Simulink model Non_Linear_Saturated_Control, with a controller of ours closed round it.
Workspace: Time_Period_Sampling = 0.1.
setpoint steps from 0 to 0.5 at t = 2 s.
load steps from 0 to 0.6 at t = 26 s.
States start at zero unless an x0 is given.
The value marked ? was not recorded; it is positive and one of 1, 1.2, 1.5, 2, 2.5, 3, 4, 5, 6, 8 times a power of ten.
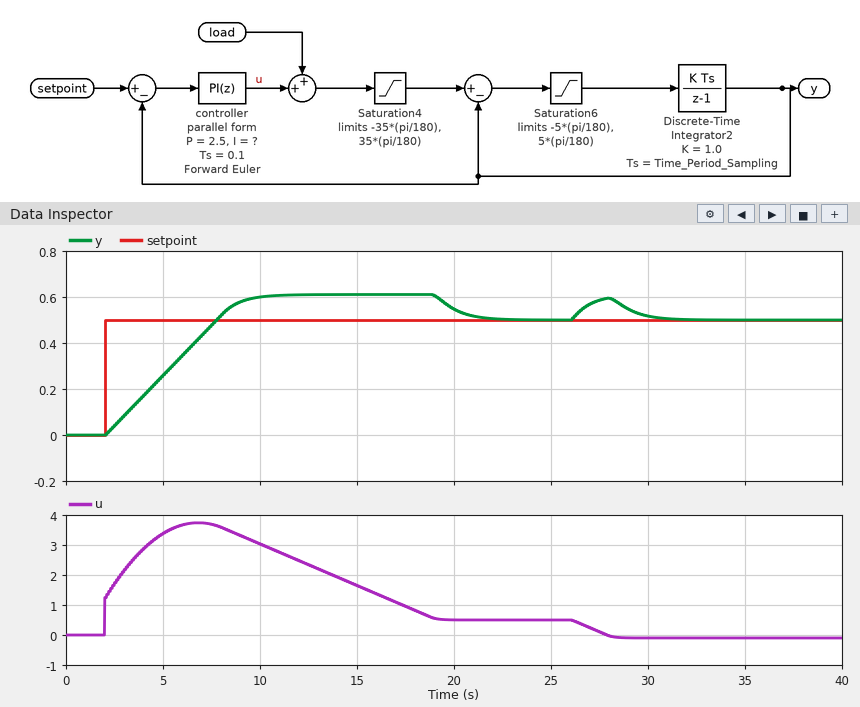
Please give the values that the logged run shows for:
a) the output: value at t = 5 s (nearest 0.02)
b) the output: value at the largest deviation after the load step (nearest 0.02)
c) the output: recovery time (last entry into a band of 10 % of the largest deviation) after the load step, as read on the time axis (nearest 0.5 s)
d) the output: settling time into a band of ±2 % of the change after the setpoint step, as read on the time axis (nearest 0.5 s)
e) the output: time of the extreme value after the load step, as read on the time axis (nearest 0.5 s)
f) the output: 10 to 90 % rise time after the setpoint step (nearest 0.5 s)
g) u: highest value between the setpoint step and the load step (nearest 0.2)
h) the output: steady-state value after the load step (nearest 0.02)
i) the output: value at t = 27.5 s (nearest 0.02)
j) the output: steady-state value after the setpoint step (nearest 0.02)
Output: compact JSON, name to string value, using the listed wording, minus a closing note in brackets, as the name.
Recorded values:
{"the output: value at t = 5 s": "0.26", "the output: value at the largest deviation after the load step": "0.60", "the output: recovery time (last entry into a band of 10 % of the largest deviation) after the load step, as read on the time axis": "30.5 s", "the output: settling time into a band of ±2 % of the change after the setpoint step, as read on the time axis": "21.5 s", "the output: time of the extreme value after the load step, as read on the time axis": "28.0 s", "the output: 10 to 90 % rise time after the setpoint step": "4.5 s", "u: highest value between the setpoint step and the load step": "3.8", "the output: steady-state value after the load step": "0.50", "the output: value at t = 27.5 s": "0.58", "the output: steady-state value after the setpoint step": "0.50"}
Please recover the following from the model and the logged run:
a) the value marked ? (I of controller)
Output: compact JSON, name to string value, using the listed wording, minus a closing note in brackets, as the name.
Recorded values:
{"the value marked ?": "2.5"}
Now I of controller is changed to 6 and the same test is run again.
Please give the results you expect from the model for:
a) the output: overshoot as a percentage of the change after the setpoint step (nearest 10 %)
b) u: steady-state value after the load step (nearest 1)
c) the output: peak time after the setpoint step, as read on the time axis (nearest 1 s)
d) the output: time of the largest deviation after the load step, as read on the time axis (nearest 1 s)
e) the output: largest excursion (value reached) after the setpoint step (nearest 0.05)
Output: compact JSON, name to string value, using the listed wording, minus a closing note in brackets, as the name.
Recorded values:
{"the output: overshoot as a percentage of the change after the setpoint step": "20 %", "u: steady-state value after the load step": "0", "the output: peak time after the setpoint step, as read on the time axis": "21 s", "the output: time of the largest deviation after the load step, as read on the time axis": "27 s", "the output: largest excursion (value reached) after the setpoint step": "0.60"}
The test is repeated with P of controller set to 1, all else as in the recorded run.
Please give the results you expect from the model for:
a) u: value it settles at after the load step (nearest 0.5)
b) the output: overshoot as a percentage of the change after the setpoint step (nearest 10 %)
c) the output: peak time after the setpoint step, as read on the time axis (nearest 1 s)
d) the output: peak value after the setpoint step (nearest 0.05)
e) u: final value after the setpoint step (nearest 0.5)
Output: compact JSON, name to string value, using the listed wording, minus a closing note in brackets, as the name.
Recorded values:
{"u: value it settles at after the load step": "0.0", "the output: overshoot as a percentage of the change after the setpoint step": "20 %", "the output: peak time after the setpoint step, as read on the time axis": "19 s", "the output: peak value after the setpoint step": "0.60", "u: final value after the setpoint step": "0.5"}
